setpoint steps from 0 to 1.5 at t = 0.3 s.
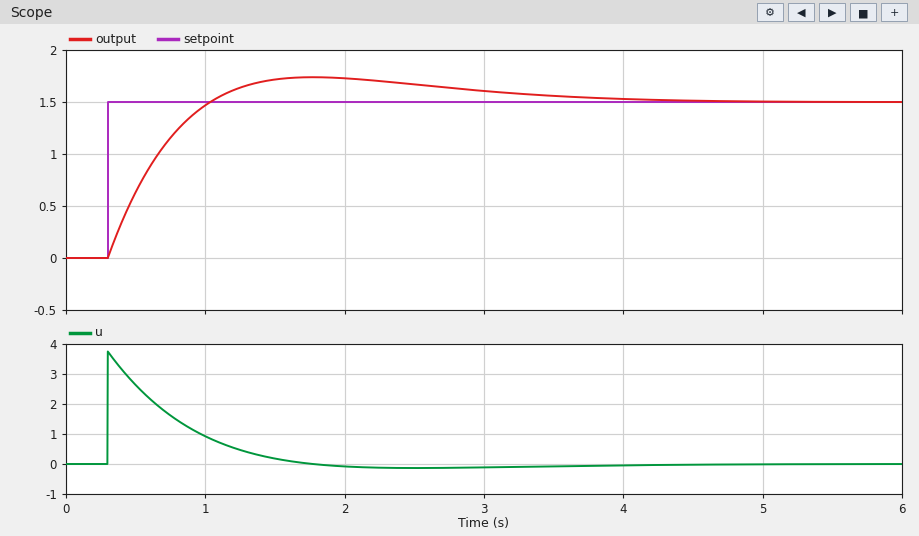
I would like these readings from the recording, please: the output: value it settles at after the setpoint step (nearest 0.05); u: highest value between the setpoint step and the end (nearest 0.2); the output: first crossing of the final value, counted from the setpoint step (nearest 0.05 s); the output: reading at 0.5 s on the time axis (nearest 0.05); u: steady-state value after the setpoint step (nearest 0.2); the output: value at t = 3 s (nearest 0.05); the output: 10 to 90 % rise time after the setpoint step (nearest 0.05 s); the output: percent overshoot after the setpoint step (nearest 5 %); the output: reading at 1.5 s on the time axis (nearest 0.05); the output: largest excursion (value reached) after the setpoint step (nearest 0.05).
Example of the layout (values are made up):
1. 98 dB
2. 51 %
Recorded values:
1. 1.50
2. 3.8
3. 0.75 s
4. 0.65
5. 0.0
6. 1.60
7. 0.55 s
8. 15 %
9. 1.70
10. 1.75
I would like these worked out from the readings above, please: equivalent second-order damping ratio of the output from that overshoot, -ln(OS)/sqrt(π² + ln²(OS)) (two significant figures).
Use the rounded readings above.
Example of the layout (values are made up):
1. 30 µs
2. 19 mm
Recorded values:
1. 0.52
